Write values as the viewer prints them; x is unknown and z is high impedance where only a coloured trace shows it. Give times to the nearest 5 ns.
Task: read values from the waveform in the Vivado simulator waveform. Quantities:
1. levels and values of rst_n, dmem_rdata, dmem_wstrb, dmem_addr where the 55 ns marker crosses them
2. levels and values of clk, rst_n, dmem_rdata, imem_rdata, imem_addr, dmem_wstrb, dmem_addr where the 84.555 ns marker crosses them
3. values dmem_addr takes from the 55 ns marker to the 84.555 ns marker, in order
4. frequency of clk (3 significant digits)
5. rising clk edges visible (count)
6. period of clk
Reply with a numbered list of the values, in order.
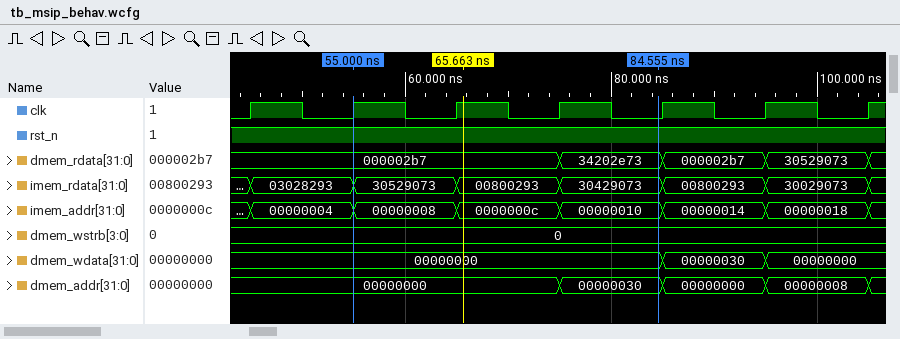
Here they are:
1. rst_n=1, dmem_rdata=000002b7, dmem_wstrb=0, dmem_addr=00000000
2. clk=0, rst_n=1, dmem_rdata=34202e73, imem_rdata=30429073, imem_addr=00000010, dmem_wstrb=0, dmem_addr=00000030
3. 00000000, 00000030
4. 100 MHz
5. 7
6. 10 ns
